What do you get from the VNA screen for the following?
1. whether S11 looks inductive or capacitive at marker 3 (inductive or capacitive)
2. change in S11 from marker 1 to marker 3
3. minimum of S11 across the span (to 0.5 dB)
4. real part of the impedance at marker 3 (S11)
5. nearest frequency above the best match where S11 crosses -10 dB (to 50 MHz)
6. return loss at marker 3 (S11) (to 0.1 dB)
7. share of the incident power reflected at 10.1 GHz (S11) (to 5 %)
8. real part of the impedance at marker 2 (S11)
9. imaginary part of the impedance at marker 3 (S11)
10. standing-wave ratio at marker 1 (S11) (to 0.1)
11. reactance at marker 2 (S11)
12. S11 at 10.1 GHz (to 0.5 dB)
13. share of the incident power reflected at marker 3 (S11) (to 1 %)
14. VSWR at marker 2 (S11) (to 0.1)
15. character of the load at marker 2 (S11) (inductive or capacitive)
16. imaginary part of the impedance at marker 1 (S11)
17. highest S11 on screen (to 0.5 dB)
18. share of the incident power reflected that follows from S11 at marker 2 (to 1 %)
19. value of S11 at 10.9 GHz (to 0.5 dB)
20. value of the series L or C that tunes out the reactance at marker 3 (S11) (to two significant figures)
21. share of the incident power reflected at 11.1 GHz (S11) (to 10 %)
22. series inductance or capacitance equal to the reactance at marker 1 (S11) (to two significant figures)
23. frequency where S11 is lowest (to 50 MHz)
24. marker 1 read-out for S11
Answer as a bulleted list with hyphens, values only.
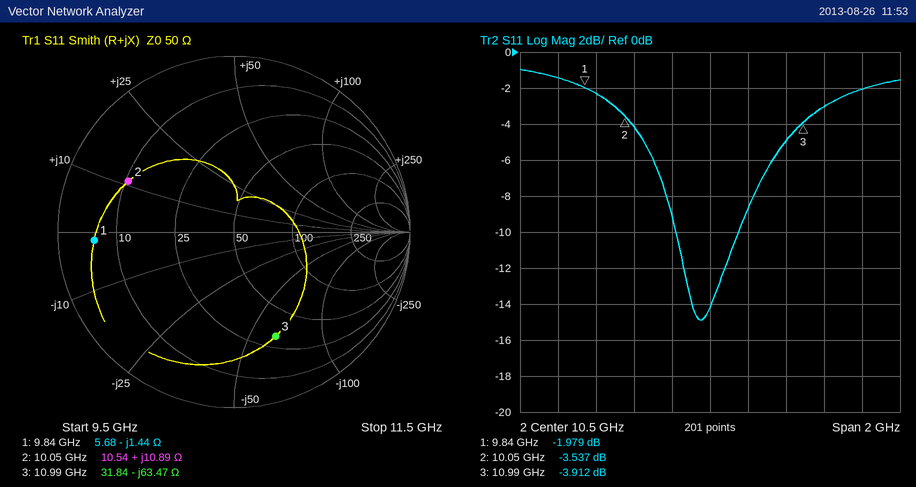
- capacitive
- -1.933 dB
- -15.0 dB
- 31.84 Ω
- 10.65 GHz
- 3.9 dB
- 40 %
- 10.54 Ω
- -63.47 Ω
- 8.8
- +10.89 Ω
- -4.0 dB
- 41 %
- 5.0
- inductive
- -1.44 Ω
- -1.0 dB
- 44 %
- -5.0 dB
- 920 pH
- 50 %
- 11 pF
- 10.45 GHz
- -1.979 dB
